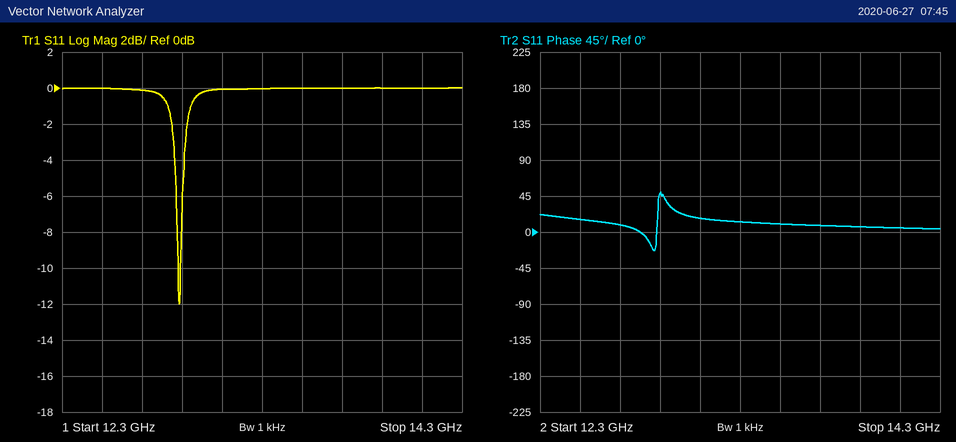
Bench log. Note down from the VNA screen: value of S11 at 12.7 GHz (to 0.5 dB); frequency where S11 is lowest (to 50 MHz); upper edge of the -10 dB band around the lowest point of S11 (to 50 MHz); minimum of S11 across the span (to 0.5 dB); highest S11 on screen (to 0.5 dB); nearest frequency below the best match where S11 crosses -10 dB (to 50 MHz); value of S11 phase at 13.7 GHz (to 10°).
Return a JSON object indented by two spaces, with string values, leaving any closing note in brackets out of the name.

{
  "value of S11 at 12.7 GHz": "0.0 dB",
  "frequency where S11 is lowest": "12.90 GHz",
  "upper edge of the -10 dB band around the lowest point of S11": "12.90 GHz",
  "minimum of S11 across the span": "-12.0 dB",
  "highest S11 on screen": "0.0 dB",
  "nearest frequency below the best match where S11 crosses -10 dB": "12.90 GHz",
  "value of S11 phase at 13.7 GHz": "10°"
}
